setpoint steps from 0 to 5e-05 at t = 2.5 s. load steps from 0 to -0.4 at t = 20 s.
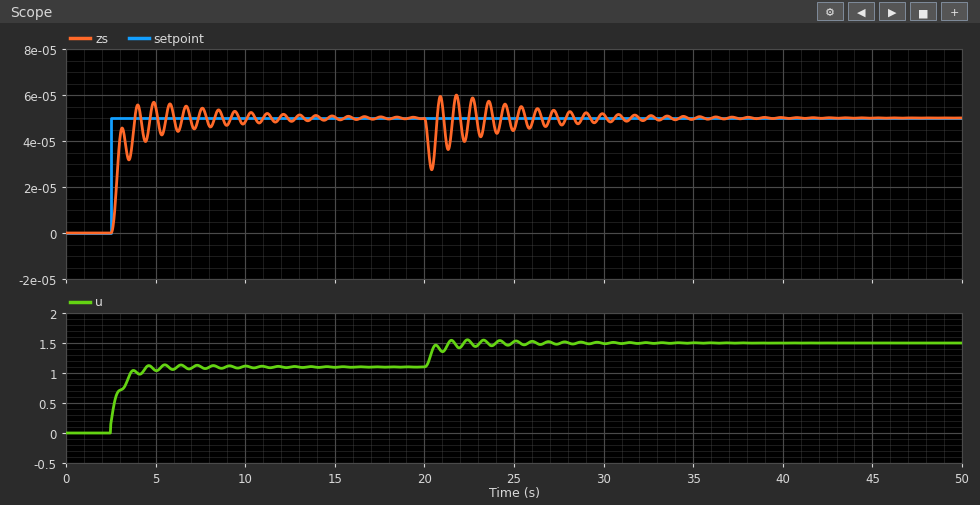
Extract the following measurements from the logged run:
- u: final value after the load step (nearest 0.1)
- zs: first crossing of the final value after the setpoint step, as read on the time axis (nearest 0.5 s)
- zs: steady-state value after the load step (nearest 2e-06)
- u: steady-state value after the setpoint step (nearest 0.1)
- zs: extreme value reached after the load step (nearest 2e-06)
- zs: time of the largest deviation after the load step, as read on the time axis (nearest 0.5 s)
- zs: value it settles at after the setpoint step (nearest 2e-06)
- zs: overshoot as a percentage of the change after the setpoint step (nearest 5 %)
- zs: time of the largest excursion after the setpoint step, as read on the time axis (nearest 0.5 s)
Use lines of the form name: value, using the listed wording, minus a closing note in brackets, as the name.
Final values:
u: final value after the load step: 1.5
zs: first crossing of the final value after the setpoint step, as read on the time axis: 4.0 s
zs: steady-state value after the load step: 0.000050
u: steady-state value after the setpoint step: 1.1
zs: extreme value reached after the load step: 0.000028
zs: time of the largest deviation after the load step, as read on the time axis: 20.5 s
zs: value it settles at after the setpoint step: 0.000050
zs: overshoot as a percentage of the change after the setpoint step: 15 %
zs: time of the largest excursion after the setpoint step, as read on the time axis: 5.0 s
